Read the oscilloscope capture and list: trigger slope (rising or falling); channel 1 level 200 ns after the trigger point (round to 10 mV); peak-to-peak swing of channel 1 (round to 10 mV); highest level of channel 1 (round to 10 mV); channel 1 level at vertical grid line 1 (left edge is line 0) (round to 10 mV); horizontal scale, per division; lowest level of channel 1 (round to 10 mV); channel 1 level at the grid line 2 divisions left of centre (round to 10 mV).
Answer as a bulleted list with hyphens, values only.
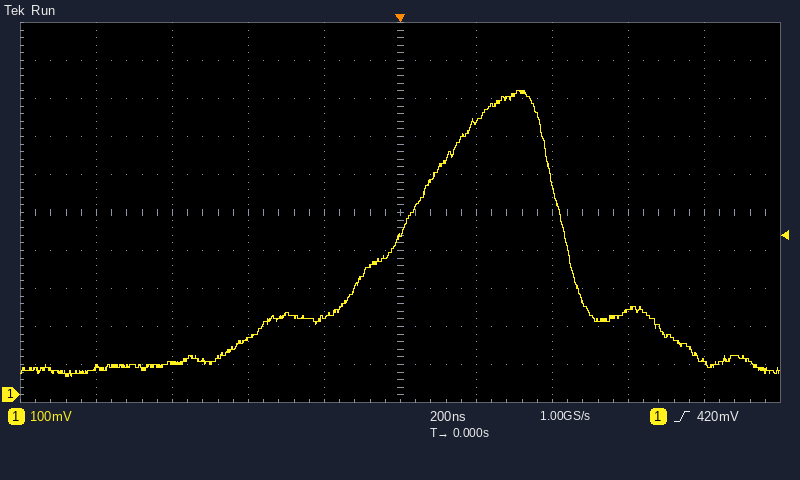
- rising
- 720 mV
- 750 mV
- 800 mV
- 70 mV
- 200 ns
- 50 mV
- 150 mV
